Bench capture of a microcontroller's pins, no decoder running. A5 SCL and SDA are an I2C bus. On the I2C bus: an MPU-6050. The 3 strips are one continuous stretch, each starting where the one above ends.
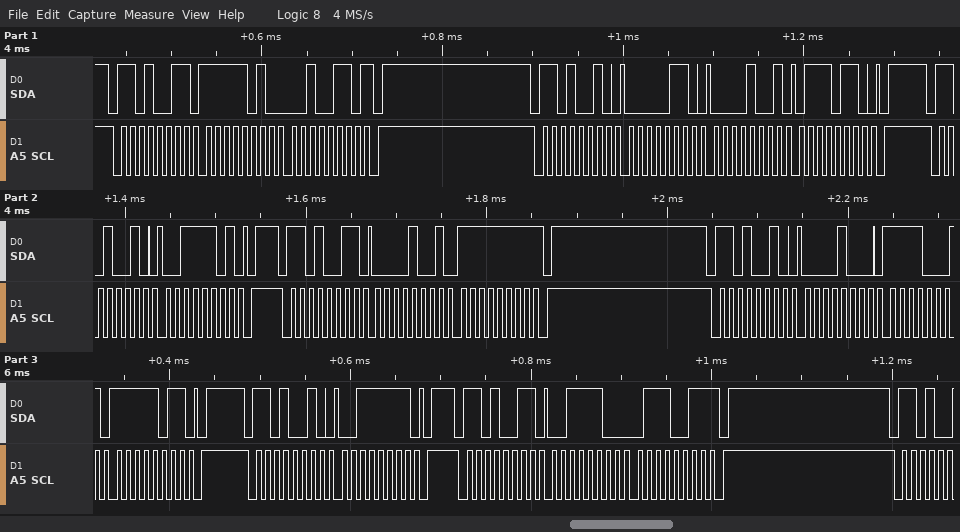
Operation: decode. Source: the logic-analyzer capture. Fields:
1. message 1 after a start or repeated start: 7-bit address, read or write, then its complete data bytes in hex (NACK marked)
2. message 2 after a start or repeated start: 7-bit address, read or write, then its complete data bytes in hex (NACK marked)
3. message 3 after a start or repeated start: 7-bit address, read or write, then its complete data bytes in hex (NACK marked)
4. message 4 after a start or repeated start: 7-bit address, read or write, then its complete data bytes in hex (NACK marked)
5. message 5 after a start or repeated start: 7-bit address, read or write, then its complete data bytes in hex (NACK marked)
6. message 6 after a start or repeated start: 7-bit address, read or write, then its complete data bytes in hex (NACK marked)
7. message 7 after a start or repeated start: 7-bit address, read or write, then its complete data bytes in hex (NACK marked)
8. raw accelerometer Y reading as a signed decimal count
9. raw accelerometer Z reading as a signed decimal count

0x69 read: FA 26 NACK
0x69 write: 06 09 76
0x69 write: 3D
0x69 read: 09 FF NACK
0x69 write: 08 F1 FB
0x69 write: 3F
0x69 read: 3C 73 NACK
2559
15475
